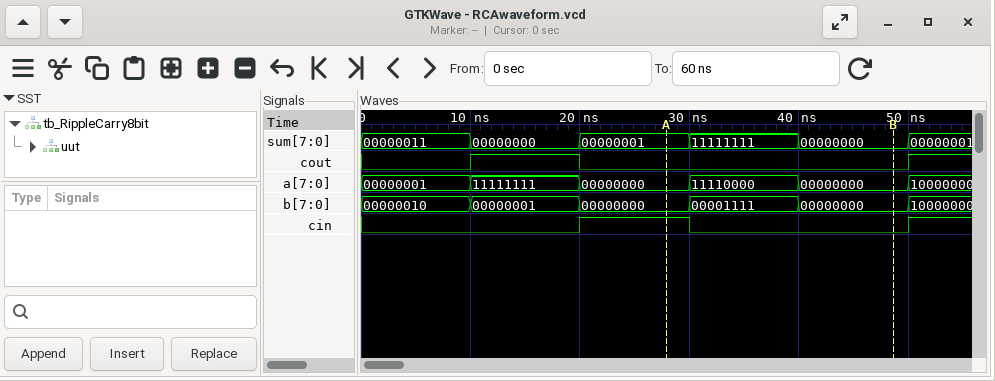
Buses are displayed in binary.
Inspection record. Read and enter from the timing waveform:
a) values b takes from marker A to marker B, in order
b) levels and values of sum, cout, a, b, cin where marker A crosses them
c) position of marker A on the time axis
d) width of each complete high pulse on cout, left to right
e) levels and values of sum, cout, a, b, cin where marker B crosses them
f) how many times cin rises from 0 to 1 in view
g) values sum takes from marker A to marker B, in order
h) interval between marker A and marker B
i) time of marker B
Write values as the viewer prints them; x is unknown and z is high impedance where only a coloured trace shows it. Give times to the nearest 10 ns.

00000000, 00001111, 00000000
sum=00000001, cout=0, a=00000000, b=00000000, cin=1
30 ns
10 ns
sum=00000000, cout=0, a=00000000, b=00000000, cin=0
2
00000001, 11111111, 00000000
20 ns
50 ns
